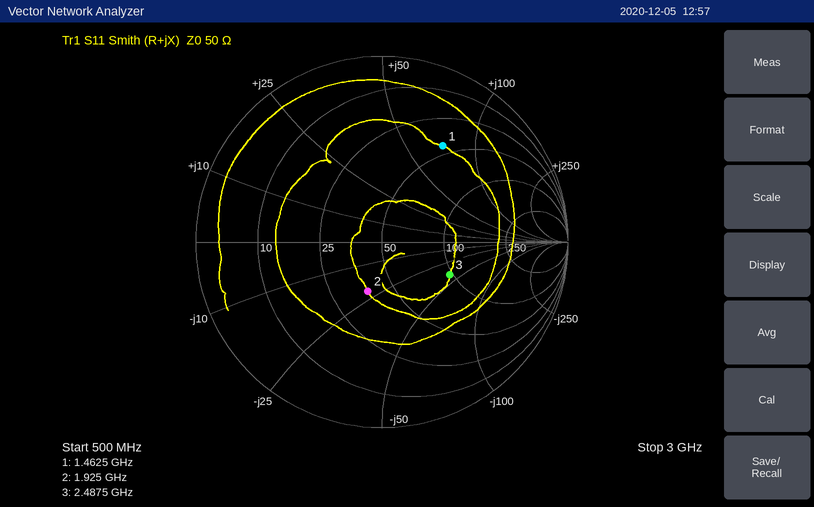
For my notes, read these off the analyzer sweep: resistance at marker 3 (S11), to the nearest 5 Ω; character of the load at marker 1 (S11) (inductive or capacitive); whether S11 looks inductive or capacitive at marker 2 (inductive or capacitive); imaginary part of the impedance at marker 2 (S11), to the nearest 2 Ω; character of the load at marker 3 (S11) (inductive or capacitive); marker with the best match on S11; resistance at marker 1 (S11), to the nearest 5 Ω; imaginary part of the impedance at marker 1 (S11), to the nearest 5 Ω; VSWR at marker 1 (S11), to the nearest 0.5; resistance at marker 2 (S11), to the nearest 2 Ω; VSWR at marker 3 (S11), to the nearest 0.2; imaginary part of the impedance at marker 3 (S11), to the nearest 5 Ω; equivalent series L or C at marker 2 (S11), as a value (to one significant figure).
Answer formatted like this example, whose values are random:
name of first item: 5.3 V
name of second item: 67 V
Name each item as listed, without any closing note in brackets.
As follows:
resistance at marker 3 (S11), to the nearest 5 Ω: 95 Ω
character of the load at marker 1 (S11): inductive
whether S11 looks inductive or capacitive at marker 2: capacitive
imaginary part of the impedance at marker 2 (S11), to the nearest 2 Ω: -22 Ω
character of the load at marker 3 (S11): capacitive
marker with the best match on S11: marker 2
resistance at marker 1 (S11), to the nearest 5 Ω: 45 Ω
imaginary part of the impedance at marker 1 (S11), to the nearest 5 Ω: +70 Ω
VSWR at marker 1 (S11), to the nearest 0.5: 4.0
resistance at marker 2 (S11), to the nearest 2 Ω: 38 Ω
VSWR at marker 3 (S11), to the nearest 0.2: 2.4
imaginary part of the impedance at marker 3 (S11), to the nearest 5 Ω: -40 Ω
equivalent series L or C at marker 2 (S11), as a value: 4 pF
